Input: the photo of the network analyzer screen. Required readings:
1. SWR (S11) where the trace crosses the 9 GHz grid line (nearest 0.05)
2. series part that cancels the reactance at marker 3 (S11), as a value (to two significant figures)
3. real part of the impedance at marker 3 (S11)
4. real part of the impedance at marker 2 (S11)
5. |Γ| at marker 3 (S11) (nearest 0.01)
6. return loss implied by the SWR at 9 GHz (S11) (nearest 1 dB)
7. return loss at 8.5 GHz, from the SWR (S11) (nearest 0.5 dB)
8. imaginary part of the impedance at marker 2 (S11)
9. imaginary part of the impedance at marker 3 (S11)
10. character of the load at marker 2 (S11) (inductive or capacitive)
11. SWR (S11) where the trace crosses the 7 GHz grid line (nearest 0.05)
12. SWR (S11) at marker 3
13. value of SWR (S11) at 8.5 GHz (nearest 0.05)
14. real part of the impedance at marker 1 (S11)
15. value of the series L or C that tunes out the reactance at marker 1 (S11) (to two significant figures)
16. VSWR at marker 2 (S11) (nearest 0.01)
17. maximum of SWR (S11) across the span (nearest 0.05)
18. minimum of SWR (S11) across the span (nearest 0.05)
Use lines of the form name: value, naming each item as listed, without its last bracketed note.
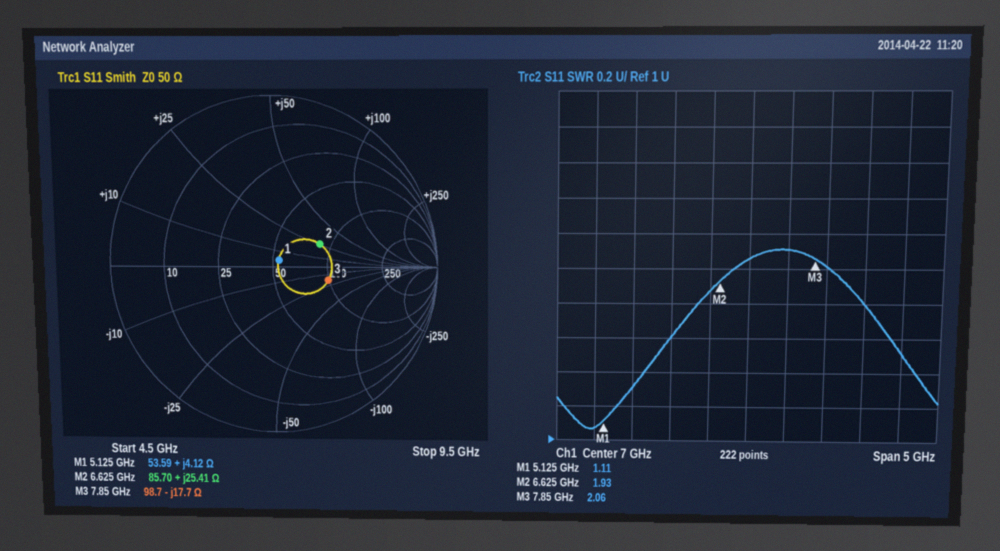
SWR (S11) where the trace crosses the 9 GHz grid line: 1.50
series part that cancels the reactance at marker 3 (S11), as a value: 360 pH
real part of the impedance at marker 3: 98.7 Ω
real part of the impedance at marker 2: 85.70 Ω
|Γ| at marker 3 (S11): 0.35
return loss implied by the SWR at 9 GHz (S11): 14 dB
return loss at 8.5 GHz, from the SWR (S11): 11.0 dB
imaginary part of the impedance at marker 2: +25.41 Ω
imaginary part of the impedance at marker 3: -17.7 Ω
character of the load at marker 2 (S11): inductive
SWR (S11) where the trace crosses the 7 GHz grid line: 2.05
SWR (S11) at marker 3: 2.06
value of SWR (S11) at 8.5 GHz: 1.80
real part of the impedance at marker 1: 53.59 Ω
value of the series L or C that tunes out the reactance at marker 1 (S11): 7.5 pF
VSWR at marker 2 (S11): 1.93
maximum of SWR (S11) across the span: 2.10
minimum of SWR (S11) across the span: 1.05
